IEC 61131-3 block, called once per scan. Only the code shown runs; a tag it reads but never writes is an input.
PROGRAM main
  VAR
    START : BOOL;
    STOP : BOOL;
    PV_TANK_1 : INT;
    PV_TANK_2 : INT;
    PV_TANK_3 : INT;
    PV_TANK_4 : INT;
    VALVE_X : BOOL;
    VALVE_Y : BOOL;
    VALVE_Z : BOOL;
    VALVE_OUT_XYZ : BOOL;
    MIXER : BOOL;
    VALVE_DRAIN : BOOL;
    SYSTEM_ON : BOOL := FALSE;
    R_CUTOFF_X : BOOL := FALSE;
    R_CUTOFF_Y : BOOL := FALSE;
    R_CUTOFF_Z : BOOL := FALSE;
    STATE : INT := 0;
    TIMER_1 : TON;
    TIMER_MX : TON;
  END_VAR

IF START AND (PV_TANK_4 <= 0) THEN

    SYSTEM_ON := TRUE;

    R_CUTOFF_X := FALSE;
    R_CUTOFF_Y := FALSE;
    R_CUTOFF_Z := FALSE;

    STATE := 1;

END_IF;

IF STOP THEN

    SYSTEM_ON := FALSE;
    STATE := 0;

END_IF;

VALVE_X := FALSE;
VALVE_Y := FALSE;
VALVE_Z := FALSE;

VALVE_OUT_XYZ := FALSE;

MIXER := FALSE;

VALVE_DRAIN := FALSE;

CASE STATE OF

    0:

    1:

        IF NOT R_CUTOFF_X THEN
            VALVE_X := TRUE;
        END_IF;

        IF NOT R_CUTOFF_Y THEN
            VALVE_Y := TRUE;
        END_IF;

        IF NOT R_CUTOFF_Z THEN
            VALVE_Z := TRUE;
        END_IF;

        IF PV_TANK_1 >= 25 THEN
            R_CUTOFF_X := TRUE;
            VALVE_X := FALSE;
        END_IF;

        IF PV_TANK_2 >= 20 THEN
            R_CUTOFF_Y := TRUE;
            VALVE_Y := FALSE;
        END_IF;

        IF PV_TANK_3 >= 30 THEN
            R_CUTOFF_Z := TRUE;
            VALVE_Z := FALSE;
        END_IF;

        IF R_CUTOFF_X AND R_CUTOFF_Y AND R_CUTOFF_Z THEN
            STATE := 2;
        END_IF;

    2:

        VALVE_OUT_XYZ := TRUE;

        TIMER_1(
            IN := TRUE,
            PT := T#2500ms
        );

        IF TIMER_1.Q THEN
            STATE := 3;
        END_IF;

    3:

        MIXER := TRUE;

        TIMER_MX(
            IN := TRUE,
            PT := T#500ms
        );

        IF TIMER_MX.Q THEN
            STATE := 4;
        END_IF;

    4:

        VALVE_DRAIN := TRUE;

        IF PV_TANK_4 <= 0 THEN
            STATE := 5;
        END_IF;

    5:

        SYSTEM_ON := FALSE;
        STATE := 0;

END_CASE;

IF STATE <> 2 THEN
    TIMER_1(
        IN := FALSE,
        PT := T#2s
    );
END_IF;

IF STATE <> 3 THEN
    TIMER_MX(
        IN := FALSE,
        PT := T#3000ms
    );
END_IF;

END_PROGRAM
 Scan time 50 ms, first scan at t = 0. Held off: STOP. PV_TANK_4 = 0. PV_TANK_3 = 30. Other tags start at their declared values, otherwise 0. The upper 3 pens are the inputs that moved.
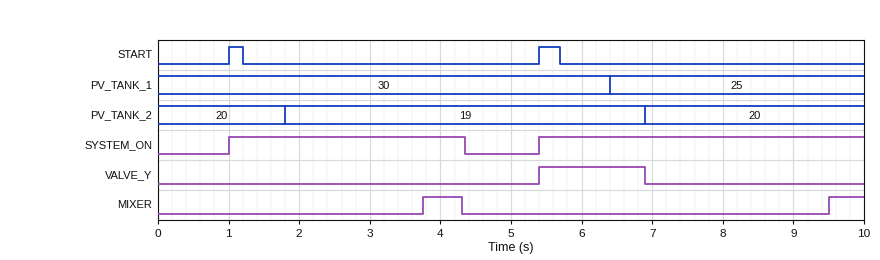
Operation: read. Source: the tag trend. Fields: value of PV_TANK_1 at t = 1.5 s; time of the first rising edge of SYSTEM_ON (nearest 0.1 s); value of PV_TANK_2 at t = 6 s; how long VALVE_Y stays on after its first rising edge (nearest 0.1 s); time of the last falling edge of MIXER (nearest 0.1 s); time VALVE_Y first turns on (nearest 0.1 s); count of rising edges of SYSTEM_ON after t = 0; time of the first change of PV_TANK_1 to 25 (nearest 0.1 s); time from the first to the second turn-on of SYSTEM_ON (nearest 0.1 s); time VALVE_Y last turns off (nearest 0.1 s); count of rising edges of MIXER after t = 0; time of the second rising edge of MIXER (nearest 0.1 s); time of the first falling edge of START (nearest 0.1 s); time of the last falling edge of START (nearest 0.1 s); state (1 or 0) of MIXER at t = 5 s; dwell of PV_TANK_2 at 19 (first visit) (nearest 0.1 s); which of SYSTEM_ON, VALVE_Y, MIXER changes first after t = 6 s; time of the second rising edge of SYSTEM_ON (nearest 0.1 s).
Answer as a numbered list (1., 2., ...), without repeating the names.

1. 30
2. 1.0 s
3. 19
4. 1.5 s
5. 4.3 s
6. 5.4 s
7. 2
8. 6.4 s
9. 4.4 s
10. 6.9 s
11. 2
12. 9.5 s
13. 1.2 s
14. 5.7 s
15. 0
16. 5.1 s
17. VALVE_Y
18. 5.4 s
